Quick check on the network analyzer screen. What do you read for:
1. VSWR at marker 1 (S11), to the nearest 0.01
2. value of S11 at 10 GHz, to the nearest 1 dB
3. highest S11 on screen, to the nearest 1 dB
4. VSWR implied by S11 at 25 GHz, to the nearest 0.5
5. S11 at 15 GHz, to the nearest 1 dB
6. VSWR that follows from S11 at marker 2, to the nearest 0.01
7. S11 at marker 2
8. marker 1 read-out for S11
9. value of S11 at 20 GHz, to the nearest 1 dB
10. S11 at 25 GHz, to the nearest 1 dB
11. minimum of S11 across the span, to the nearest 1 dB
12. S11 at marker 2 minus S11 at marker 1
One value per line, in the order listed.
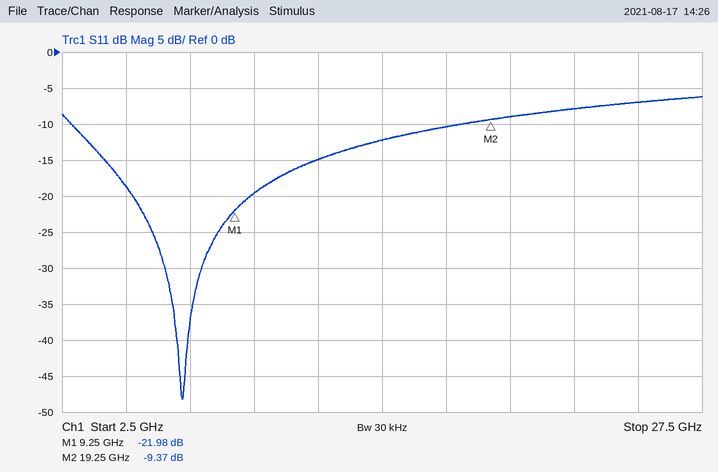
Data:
1.17
-20 dB
-6 dB
2.5
-12 dB
2.03
-9.37 dB
-21.98 dB
-9 dB
-7 dB
-48 dB
12.61 dB
